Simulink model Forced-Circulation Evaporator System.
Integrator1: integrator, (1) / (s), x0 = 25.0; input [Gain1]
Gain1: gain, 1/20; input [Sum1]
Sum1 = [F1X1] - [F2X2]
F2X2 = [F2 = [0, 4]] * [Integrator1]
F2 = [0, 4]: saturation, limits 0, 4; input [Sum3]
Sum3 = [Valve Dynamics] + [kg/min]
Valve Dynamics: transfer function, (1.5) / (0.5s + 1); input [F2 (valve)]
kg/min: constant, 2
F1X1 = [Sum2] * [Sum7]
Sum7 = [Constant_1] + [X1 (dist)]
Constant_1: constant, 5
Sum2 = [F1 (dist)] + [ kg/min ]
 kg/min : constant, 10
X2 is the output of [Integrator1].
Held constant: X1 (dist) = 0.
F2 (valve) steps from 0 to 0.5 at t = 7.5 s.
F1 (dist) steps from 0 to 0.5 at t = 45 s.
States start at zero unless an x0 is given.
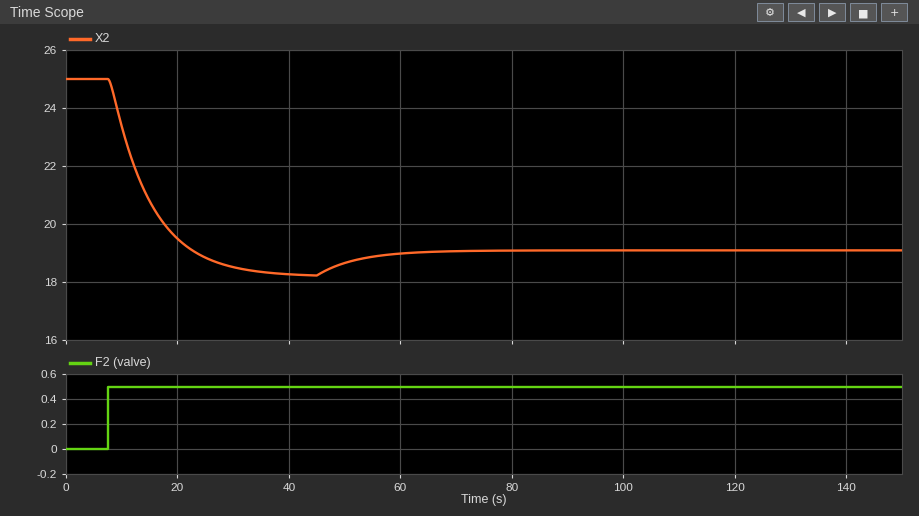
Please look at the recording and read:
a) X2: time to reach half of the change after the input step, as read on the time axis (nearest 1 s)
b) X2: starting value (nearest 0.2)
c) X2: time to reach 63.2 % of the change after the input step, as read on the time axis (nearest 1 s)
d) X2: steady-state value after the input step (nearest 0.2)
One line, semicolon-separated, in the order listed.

13 s; 25.0; 15 s; 18.2
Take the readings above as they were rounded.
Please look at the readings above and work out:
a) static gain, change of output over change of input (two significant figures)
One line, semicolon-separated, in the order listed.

-14
